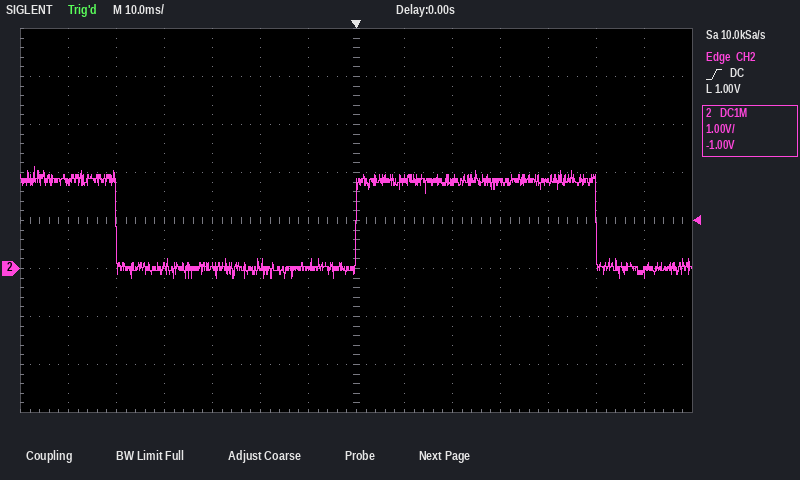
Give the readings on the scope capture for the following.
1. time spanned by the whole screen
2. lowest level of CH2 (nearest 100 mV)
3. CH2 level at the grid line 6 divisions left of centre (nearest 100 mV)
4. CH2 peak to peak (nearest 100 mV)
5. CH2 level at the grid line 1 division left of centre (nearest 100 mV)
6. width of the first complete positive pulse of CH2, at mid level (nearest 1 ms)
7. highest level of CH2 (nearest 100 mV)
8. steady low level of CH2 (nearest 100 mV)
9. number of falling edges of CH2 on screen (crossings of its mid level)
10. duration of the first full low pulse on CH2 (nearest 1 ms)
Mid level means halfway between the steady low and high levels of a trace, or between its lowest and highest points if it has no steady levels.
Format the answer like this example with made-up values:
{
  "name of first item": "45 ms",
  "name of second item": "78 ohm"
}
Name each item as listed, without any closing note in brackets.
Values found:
{
  "time spanned by the whole screen": "140 ms",
  "lowest level of CH2": "-200 mV",
  "CH2 level at the grid line 6 divisions left of centre": "1.8 V",
  "CH2 peak to peak": "2.3 V",
  "CH2 level at the grid line 1 division left of centre": "0.0 V",
  "width of the first complete positive pulse of CH2, at mid level": "50 ms",
  "highest level of CH2": "2.1 V",
  "steady low level of CH2": "0.0 V",
  "number of falling edges of CH2 on screen": "2",
  "duration of the first full low pulse on CH2": "50 ms"
}
